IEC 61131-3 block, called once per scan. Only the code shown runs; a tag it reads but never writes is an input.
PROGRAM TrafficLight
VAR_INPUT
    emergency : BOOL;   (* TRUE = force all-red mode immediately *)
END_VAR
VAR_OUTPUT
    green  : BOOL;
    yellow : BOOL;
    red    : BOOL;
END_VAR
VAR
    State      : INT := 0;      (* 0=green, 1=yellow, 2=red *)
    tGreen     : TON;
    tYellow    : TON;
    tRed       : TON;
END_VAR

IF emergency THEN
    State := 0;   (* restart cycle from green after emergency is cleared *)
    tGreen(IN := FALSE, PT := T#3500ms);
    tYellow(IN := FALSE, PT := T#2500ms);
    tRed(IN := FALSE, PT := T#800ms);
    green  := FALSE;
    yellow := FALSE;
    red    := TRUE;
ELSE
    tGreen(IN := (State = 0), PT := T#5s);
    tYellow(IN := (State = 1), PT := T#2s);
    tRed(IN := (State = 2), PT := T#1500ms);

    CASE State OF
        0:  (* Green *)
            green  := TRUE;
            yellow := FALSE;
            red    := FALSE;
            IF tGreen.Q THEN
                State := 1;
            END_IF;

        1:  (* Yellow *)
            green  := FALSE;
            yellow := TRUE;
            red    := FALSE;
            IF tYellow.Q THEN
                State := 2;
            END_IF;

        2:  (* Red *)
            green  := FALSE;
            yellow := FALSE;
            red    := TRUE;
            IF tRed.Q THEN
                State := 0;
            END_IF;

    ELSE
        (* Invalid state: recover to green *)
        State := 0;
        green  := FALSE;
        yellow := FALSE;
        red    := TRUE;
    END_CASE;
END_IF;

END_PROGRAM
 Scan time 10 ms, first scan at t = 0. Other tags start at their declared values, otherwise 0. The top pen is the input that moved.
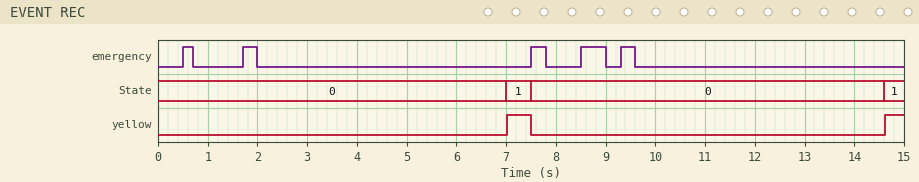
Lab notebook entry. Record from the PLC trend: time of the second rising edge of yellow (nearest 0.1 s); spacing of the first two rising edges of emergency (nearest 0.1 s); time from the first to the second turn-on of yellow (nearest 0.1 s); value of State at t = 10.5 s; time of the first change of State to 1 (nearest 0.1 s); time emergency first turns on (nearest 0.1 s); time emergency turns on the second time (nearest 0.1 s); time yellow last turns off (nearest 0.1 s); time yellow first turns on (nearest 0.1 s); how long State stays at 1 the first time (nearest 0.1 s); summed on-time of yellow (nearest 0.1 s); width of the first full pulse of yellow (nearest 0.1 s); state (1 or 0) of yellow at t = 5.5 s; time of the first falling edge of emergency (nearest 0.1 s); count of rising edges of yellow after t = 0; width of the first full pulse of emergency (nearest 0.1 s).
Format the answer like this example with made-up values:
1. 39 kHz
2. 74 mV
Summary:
1. 14.6 s
2. 1.2 s
3. 7.6 s
4. 0
5. 7.0 s
6. 0.5 s
7. 1.7 s
8. 7.5 s
9. 7.0 s
10. 0.5 s
11. 0.9 s
12. 0.5 s
13. 0
14. 0.7 s
15. 2
16. 0.2 s
